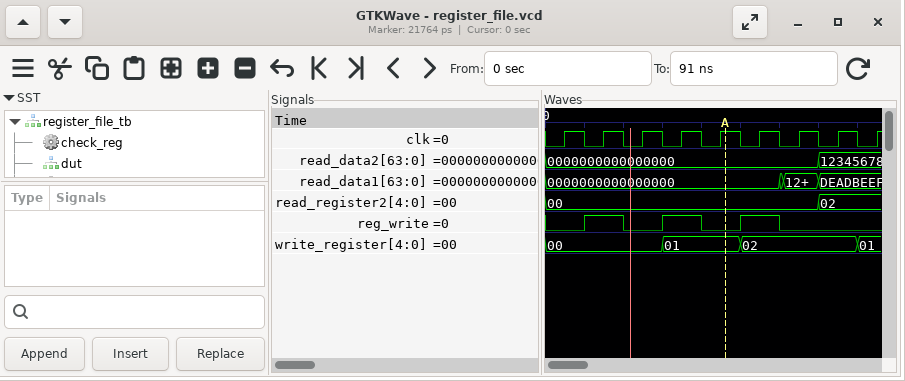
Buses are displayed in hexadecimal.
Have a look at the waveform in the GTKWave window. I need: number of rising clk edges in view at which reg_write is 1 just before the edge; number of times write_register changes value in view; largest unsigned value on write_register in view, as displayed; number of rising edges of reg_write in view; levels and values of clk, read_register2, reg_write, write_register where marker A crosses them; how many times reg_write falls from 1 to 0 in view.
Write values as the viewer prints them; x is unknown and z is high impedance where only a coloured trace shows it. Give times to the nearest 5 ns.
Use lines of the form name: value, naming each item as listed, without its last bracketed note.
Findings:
number of rising clk edges in view at which reg_write is 1 just before the edge: 3
number of times write_register changes value in view: 3
largest unsigned value on write_register in view, as displayed: 02
number of rising edges of reg_write in view: 3
levels and values of clk, read_register2, reg_write, write_register where marker A crosses them: clk=1, read_register2=00, reg_write=0, write_register=01
how many times reg_write falls from 1 to 0 in view: 3
